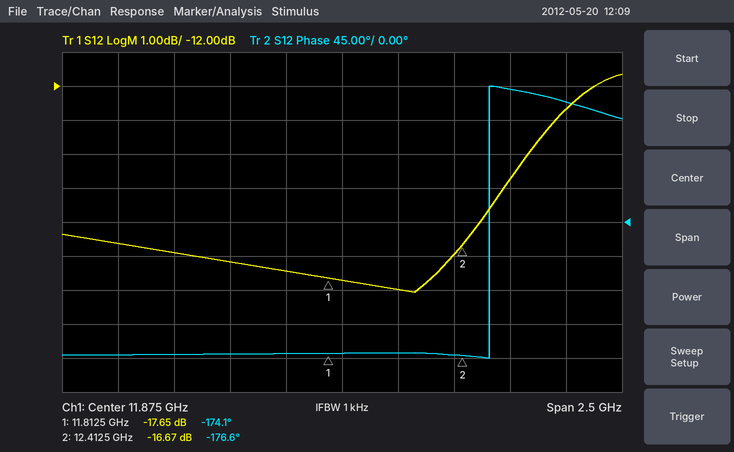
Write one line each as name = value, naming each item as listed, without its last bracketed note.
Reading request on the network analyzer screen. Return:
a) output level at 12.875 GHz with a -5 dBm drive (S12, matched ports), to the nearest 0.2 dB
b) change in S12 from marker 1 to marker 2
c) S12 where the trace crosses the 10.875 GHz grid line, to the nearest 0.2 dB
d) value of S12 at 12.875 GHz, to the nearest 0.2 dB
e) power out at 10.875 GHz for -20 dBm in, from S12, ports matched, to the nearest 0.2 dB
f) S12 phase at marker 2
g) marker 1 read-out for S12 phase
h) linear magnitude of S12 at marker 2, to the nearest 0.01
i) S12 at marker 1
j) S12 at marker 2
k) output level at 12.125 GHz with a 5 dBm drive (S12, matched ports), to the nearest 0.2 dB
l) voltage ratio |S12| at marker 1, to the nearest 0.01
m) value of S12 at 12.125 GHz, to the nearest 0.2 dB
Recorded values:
output level at 12.875 GHz with a -5 dBm drive (S12, matched ports), to the nearest 0.2 dB = -17.6 dBm
change in S12 from marker 1 to marker 2 = 0.98 dB
S12 where the trace crosses the 10.875 GHz grid line, to the nearest 0.2 dB = -16.6 dB
value of S12 at 12.875 GHz, to the nearest 0.2 dB = -12.6 dB
power out at 10.875 GHz for -20 dBm in, from S12, ports matched, to the nearest 0.2 dB = -36.6 dBm
S12 phase at marker 2 = -176.6°
marker 1 read-out for S12 phase = -174.1°
linear magnitude of S12 at marker 2, to the nearest 0.01 = 0.15
S12 at marker 1 = -17.65 dB
S12 at marker 2 = -16.67 dB
output level at 12.125 GHz with a 5 dBm drive (S12, matched ports), to the nearest 0.2 dB = -13.0 dBm
voltage ratio |S12| at marker 1, to the nearest 0.01 = 0.13
value of S12 at 12.125 GHz, to the nearest 0.2 dB = -18.0 dB
